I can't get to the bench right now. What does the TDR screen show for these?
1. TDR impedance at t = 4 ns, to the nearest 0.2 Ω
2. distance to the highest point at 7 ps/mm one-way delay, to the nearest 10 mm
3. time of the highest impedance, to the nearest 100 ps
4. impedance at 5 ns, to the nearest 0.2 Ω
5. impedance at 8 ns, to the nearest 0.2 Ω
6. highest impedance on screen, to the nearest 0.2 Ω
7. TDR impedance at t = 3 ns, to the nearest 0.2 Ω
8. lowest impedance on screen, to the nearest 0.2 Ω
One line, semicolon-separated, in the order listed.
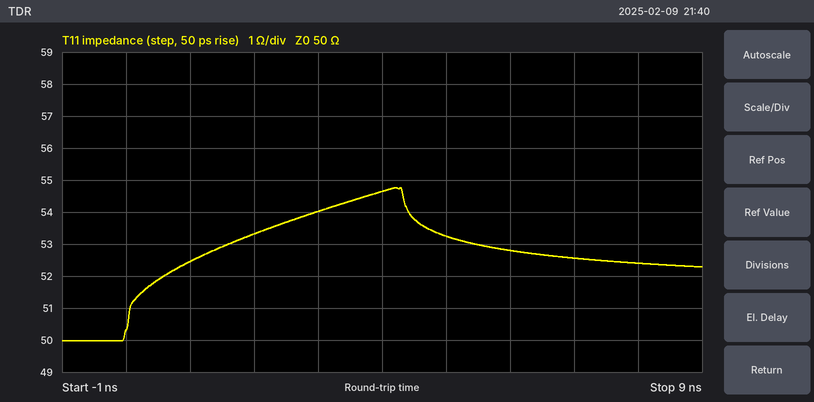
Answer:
54.6 Ω; 300 mm; 4.2 ns; 53.2 Ω; 52.4 Ω; 54.8 Ω; 54.0 Ω; 50.0 Ω
